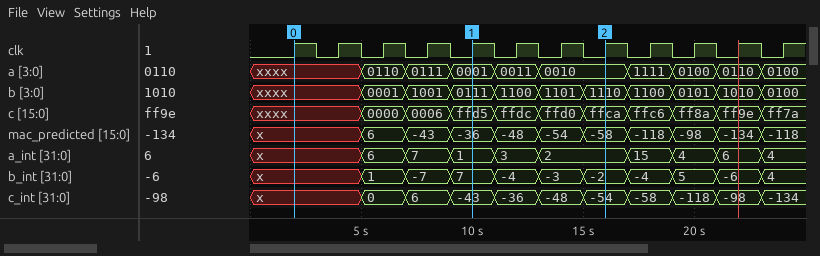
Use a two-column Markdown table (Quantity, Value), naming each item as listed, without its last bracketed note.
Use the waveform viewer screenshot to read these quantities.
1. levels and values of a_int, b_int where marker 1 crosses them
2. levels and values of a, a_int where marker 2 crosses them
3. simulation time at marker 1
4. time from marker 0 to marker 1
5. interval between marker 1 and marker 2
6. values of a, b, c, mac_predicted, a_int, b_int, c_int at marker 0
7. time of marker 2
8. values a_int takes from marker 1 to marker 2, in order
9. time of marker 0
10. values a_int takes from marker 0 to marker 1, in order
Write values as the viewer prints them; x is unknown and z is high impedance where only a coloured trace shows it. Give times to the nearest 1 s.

| Quantity | Value |
|---|---|
| levels and values of a_int, b_int where marker 1 crosses them | a_int=1, b_int=7 |
| levels and values of a, a_int where marker 2 crosses them | a=0010, a_int=2 |
| simulation time at marker 1 | 10 s |
| time from marker 0 to marker 1 | 8 s |
| interval between marker 1 and marker 2 | 6 s |
| values of a, b, c, mac_predicted, a_int, b_int, c_int at marker 0 | a=xxxx, b=xxxx, c=xxxx, mac_predicted=x, a_int=x, b_int=x, c_int=x |
| time of marker 2 | 16 s |
| values a_int takes from marker 1 to marker 2, in order | 1, 3, 2 |
| time of marker 0 | 2 s |
| values a_int takes from marker 0 to marker 1, in order | x, 6, 7, 1 |
